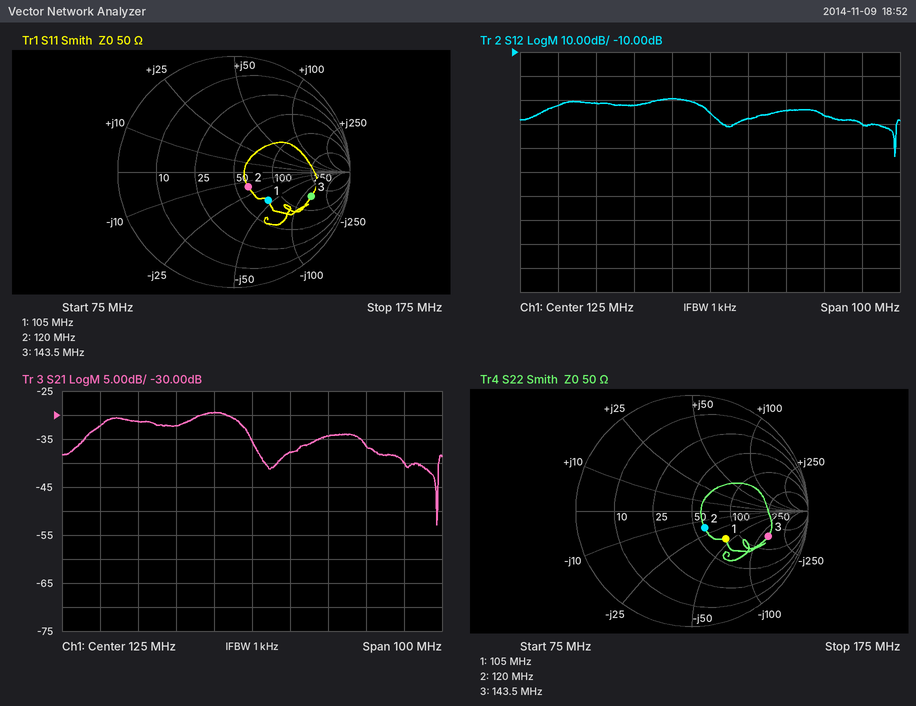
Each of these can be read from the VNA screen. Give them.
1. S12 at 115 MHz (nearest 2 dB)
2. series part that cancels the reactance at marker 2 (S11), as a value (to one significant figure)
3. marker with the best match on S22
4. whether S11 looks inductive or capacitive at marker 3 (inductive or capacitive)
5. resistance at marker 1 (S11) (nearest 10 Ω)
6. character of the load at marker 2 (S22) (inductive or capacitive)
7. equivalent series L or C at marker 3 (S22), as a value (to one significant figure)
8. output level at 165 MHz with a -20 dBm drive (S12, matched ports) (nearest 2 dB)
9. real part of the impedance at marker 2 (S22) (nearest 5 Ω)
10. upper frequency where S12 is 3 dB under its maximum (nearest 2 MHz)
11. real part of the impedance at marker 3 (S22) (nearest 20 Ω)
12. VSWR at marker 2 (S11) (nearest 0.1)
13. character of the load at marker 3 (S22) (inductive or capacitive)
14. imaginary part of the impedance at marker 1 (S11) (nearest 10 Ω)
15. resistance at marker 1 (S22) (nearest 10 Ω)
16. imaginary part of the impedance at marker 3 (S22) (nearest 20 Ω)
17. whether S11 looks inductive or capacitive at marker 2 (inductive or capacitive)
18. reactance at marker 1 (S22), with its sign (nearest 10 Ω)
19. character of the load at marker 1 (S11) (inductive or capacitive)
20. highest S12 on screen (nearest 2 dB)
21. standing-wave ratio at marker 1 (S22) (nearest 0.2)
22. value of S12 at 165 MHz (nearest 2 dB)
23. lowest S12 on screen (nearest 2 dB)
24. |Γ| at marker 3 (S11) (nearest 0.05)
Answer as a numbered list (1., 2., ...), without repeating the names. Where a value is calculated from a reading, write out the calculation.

1. -30 dB
2. L = 15 Ω/(2π × 120 MHz) ≈ 20 nH
3. marker 2
4. capacitive
5. 80 Ω
6. capacitive
7. C = 1/(2π × 143.5 MHz × 140 Ω) ≈ 8 pF
8. -20 dBm + (-40 dB) = -60 dBm
9. 60 Ω
10. 122 MHz
11. 160 Ω
12. 1.4
13. capacitive
14. -40 Ω
15. 80 Ω
16. -140 Ω
17. capacitive
18. -40 Ω
19. capacitive
20. -30 dB
21. 2.2
22. -40 dB
23. -54 dB
24. 0.70
